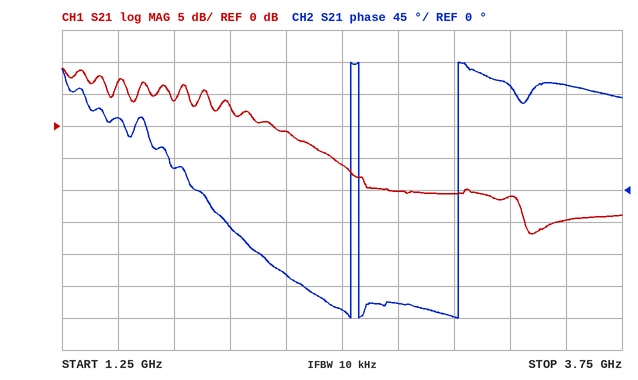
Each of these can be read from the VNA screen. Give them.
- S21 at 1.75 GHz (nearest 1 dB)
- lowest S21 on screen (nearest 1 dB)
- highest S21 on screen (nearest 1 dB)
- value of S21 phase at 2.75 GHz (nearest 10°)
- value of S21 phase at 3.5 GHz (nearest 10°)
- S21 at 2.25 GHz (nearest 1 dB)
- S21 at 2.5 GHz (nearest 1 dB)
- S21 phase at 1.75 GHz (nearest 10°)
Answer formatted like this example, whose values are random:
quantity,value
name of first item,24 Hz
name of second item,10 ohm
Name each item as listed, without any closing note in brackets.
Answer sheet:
quantity,value
S21 at 1.75 GHz,4 dB
lowest S21 on screen,-17 dB
highest S21 on screen,9 dB
value of S21 phase at 2.75 GHz,-160°
value of S21 phase at 3.5 GHz,150°
S21 at 2.25 GHz,-1 dB
S21 at 2.5 GHz,-6 dB
S21 phase at 1.75 GHz,30°
